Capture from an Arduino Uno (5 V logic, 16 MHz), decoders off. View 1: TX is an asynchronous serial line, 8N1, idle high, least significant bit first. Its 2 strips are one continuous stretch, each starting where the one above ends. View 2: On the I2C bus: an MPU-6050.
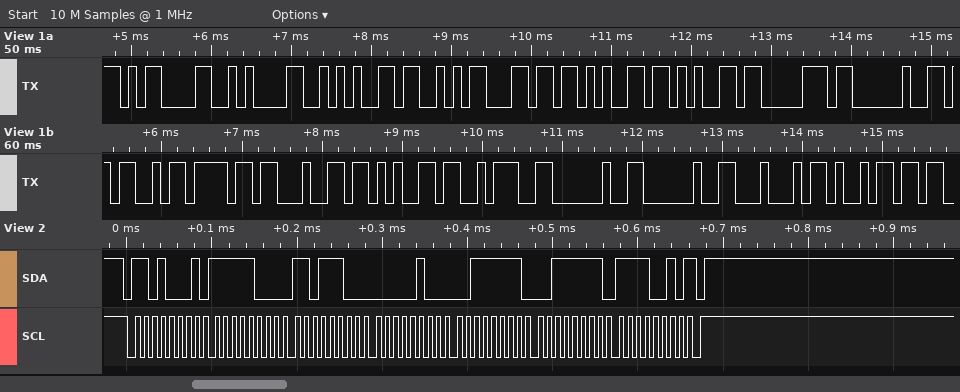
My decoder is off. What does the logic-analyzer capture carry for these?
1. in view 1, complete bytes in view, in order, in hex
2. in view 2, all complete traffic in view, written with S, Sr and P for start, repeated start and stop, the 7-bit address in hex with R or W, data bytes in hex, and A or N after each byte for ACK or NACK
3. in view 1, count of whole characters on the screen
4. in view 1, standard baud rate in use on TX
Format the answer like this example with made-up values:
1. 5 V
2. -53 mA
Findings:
1. 0D 0A 2A 53 6C 65 65 70 20 4D 6F 64 65 3A 20 20 44 69
2. S 68R A F8 A DC A 04 A 3F A 3F A F2 N P
3. 18
4. 9600 baud
